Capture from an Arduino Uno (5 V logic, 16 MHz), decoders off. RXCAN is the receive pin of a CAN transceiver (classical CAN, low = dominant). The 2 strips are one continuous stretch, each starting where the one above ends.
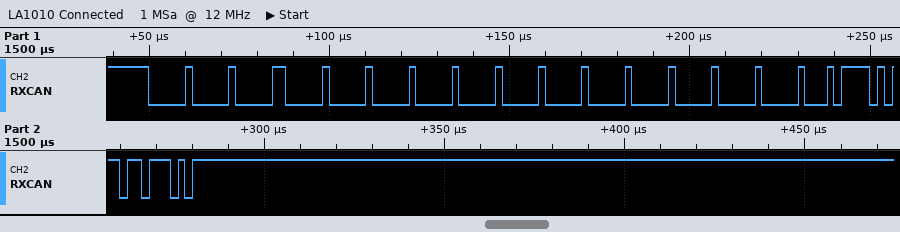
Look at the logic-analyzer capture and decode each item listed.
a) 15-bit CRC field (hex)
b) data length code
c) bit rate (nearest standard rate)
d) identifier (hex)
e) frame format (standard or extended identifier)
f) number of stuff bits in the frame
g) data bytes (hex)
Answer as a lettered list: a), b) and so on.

a) 0x6B6E
b) 8
c) 500 kbit/s
d) 0x000
e) standard
f) 15
g) 00 00 00 00 00 00 00 0B
